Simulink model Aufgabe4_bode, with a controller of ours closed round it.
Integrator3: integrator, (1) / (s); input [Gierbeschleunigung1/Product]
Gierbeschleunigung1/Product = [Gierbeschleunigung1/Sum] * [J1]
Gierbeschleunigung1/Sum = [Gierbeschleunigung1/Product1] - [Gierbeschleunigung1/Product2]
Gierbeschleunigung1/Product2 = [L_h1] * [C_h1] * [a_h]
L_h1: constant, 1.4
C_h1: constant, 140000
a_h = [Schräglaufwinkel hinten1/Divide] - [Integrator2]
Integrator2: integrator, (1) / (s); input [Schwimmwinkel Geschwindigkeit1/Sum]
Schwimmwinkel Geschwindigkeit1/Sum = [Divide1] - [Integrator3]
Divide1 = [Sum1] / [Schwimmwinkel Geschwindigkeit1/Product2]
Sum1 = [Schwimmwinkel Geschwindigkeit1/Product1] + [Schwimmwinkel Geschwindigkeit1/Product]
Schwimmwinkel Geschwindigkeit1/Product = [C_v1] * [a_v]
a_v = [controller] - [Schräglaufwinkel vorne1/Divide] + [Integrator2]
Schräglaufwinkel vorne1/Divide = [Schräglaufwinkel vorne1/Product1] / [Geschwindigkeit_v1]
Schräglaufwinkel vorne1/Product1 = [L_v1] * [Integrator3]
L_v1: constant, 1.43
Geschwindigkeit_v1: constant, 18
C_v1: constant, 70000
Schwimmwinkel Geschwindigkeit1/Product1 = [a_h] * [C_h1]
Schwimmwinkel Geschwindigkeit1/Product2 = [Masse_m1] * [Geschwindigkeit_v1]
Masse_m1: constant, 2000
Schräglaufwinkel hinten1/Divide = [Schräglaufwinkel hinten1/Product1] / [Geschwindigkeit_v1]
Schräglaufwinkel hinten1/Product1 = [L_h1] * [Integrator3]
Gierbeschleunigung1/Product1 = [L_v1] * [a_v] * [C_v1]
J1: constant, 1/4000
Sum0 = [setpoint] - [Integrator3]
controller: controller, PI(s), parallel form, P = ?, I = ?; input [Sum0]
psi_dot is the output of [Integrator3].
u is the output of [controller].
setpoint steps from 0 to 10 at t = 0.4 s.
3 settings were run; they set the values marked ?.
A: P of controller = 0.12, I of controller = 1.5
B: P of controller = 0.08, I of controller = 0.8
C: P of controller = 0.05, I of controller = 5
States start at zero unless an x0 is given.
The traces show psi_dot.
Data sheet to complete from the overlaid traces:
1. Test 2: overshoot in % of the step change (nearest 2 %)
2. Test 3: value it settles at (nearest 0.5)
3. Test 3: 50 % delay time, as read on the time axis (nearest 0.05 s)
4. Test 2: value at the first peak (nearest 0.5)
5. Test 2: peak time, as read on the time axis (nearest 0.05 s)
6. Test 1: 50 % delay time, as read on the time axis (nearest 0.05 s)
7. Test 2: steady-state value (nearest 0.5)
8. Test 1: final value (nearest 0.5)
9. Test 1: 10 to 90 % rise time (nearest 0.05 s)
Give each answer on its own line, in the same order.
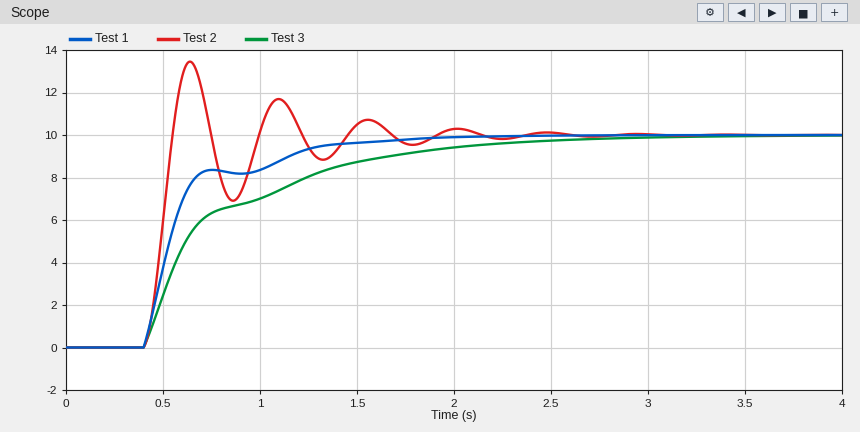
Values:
34 %
10.0
0.60 s
13.5
0.65 s
0.55 s
10.0
10.0
0.70 s
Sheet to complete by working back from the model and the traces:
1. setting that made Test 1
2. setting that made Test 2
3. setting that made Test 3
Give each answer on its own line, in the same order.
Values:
A
C
B
